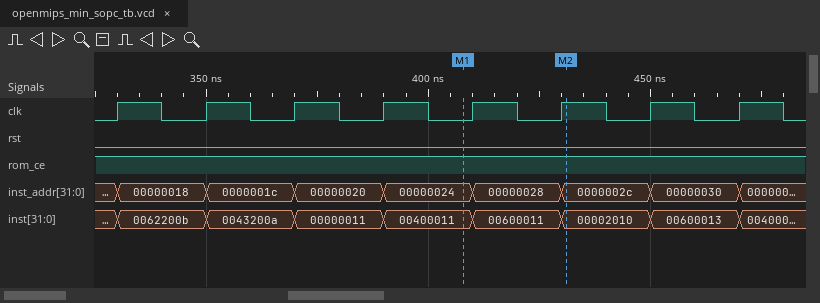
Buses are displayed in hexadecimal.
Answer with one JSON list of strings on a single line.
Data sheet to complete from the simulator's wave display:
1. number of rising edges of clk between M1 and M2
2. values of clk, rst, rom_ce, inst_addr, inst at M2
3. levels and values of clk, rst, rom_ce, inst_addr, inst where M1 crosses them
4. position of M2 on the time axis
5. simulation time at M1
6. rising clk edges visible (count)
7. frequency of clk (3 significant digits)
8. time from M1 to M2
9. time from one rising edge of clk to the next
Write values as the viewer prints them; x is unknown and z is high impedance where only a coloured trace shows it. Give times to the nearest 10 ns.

["2", "clk=1, rst=0, rom_ce=1, inst_addr=0000002c, inst=00002010", "clk=0, rst=0, rom_ce=1, inst_addr=00000024, inst=00400011", "430 ns", "410 ns", "8", "50.0 MHz", "20 ns", "20 ns"]
